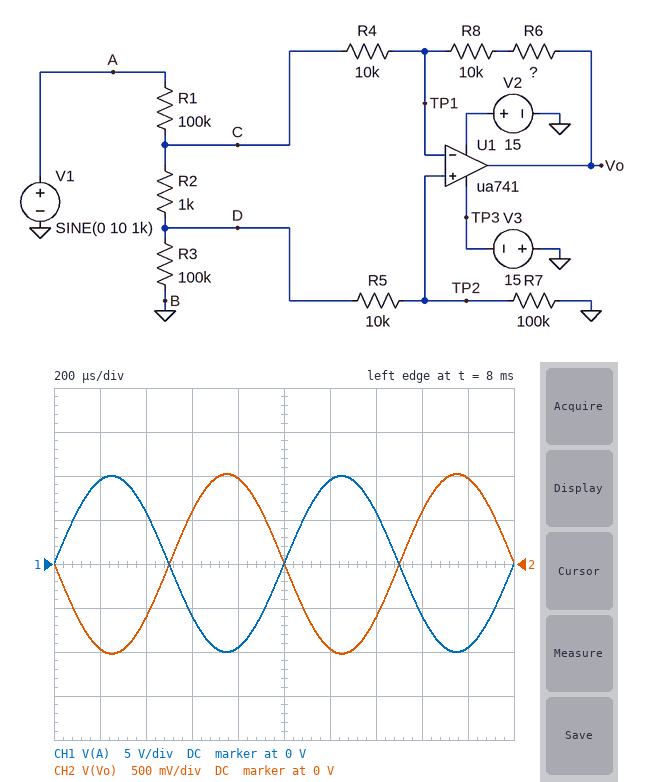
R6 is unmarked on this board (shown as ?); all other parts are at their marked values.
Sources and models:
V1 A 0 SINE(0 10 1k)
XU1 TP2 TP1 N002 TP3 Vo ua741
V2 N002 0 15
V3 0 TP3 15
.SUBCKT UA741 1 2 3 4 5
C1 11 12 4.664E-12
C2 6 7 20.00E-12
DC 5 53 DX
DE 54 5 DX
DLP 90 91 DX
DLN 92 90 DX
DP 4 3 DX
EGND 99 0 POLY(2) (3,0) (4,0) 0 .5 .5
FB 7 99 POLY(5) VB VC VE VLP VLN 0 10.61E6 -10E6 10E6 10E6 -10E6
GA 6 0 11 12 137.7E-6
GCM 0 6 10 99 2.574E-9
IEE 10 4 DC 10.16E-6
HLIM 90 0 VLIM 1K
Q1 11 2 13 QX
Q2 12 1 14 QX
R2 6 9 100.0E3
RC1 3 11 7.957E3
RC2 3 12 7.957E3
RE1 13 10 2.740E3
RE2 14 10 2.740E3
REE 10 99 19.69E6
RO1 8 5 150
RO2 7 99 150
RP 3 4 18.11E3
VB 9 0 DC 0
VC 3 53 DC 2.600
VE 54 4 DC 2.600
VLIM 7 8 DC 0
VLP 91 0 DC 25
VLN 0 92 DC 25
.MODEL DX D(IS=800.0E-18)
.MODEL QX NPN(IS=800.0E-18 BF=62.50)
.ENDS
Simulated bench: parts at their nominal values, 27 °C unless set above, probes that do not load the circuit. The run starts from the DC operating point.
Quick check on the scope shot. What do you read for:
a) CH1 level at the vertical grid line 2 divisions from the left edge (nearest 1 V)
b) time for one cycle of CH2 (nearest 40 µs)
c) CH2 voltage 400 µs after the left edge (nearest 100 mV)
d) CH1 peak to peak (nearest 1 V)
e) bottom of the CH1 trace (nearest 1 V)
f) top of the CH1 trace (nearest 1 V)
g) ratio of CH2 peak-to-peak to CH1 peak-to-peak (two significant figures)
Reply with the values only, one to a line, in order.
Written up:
6 V
1.00 ms
-600 mV
20 V
-10 V
10 V
0.10
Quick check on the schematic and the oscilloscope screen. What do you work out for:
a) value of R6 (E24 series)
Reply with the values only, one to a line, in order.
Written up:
110 kΩ
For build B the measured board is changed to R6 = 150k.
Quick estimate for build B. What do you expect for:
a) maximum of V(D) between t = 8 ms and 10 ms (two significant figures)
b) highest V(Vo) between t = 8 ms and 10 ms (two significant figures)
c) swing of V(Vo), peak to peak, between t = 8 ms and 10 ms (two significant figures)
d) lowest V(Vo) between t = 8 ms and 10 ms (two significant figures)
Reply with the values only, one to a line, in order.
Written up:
2.5 V
2.1 V
4.2 V
-2.1 V
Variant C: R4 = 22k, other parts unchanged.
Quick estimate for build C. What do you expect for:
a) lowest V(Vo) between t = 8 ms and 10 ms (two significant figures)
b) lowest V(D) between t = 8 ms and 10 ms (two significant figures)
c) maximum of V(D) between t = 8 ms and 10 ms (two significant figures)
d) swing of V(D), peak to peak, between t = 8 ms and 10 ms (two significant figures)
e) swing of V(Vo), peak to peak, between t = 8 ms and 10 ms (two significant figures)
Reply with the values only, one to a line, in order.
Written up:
-900 mV
-2.9 V
2.9 V
5.8 V
1.8 V
